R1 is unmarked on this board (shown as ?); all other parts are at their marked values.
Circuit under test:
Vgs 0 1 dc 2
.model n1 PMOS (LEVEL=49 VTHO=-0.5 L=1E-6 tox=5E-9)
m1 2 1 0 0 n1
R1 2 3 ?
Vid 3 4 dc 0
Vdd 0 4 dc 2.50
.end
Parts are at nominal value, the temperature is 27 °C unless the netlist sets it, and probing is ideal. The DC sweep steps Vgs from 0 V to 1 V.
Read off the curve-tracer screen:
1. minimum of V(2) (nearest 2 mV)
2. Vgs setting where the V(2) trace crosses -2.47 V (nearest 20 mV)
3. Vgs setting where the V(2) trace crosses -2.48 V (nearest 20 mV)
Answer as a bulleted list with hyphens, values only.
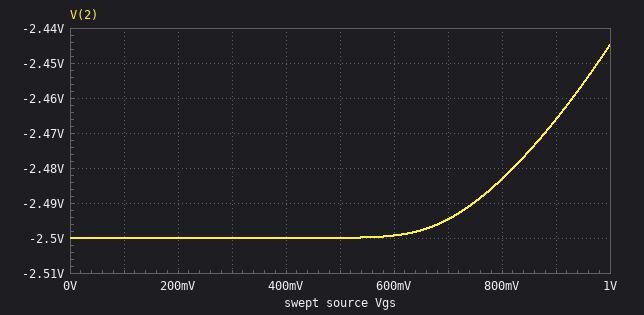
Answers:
- -2.500 V
- 880 mV
- 820 mV
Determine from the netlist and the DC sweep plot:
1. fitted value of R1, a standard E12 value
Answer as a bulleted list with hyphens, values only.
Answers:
- 1.5 kΩ
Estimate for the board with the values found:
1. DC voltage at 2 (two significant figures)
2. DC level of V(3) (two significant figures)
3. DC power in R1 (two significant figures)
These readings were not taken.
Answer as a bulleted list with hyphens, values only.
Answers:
- -2.1 V
- -2.5 V
- 120 µW
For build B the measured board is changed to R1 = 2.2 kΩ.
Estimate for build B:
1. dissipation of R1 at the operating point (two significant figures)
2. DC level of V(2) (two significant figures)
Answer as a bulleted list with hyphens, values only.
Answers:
- 180 µW
- -1.9 V
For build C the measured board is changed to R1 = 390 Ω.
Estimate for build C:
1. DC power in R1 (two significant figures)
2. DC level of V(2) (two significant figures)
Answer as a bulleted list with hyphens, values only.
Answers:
- 32 µW
- -2.4 V
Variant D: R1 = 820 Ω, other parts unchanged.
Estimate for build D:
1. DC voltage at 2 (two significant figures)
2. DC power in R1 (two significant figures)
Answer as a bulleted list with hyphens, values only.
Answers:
- -2.3 V
- 67 µW
